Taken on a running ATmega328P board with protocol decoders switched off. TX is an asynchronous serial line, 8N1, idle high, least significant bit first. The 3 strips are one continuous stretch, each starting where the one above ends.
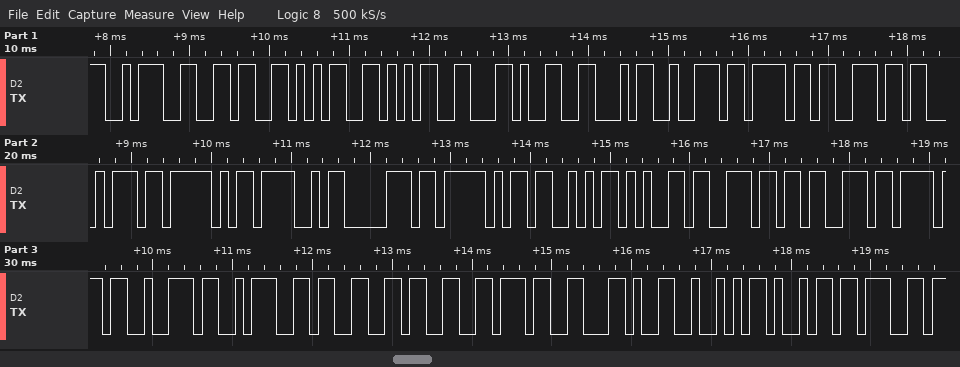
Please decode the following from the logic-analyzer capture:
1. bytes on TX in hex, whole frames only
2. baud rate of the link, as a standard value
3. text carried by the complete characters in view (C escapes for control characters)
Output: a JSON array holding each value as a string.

["3A 36 35 35 2C 46 72 6F 6E 74 5F 4F 70 5F 53 65 6E 73 6F 72 3A 33 33 37 2C 52 69 67", "9600 baud", "\":655,Front_Op_Sensor:337,Rig\""]
